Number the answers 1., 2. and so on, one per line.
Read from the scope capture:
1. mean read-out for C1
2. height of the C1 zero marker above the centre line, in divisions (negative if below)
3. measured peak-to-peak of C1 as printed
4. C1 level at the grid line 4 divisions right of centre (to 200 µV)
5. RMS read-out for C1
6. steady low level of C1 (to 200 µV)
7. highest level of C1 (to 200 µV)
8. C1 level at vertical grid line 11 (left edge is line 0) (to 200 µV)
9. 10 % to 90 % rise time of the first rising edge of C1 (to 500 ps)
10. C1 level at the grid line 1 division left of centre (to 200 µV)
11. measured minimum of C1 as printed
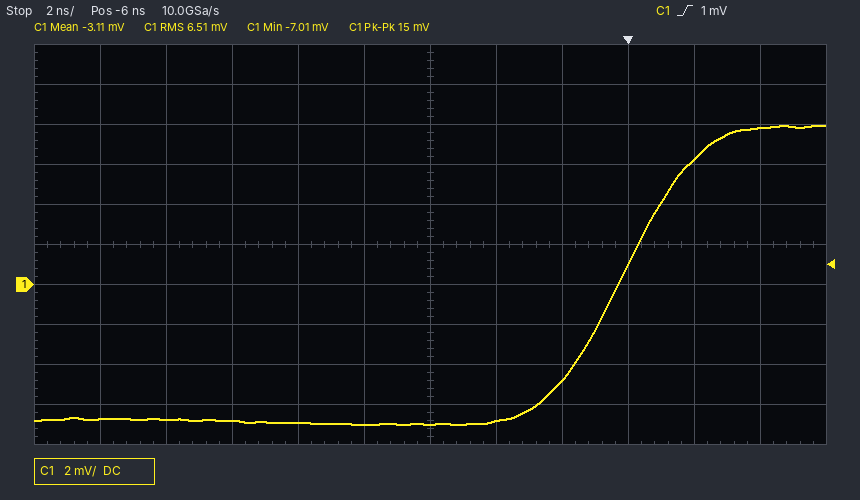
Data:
1. -3.11 mV
2. -1.0 div
3. 15 mV
4. 6.2 mV
5. 6.51 mV
6. -6.8 mV
7. 8.0 mV
8. 7.8 mV
9. 4.5 ns
10. -7.0 mV
11. -7.01 mV
